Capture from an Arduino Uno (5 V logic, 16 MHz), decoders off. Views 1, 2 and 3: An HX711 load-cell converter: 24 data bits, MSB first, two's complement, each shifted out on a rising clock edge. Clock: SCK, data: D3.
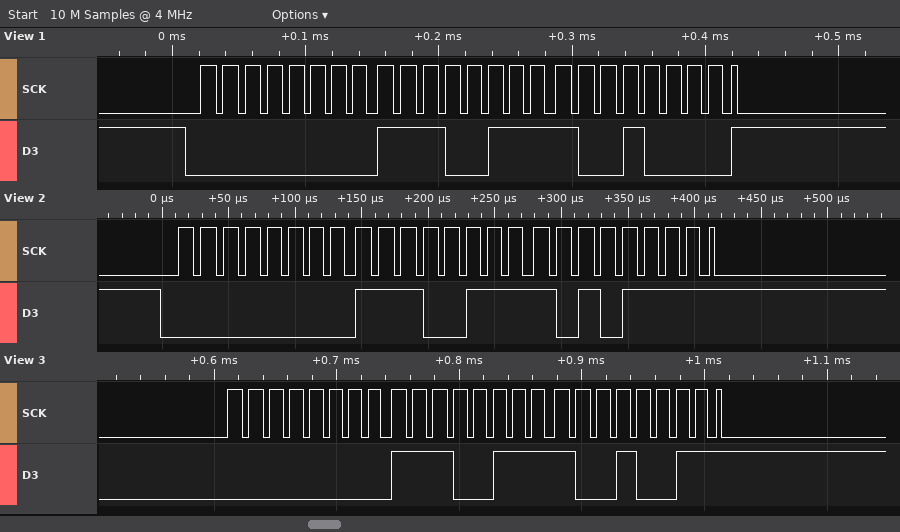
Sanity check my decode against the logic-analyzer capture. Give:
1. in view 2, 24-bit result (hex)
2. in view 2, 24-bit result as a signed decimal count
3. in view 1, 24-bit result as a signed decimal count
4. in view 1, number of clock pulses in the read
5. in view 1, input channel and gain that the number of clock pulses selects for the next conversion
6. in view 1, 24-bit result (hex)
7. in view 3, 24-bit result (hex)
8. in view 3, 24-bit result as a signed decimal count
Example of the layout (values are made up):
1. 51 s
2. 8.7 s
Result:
1. 0x00E7AF
2. 59311
3. 59280
4. 25
5. channel A, gain 128
6. 0x00E790
7. 0x00E793
8. 59283
